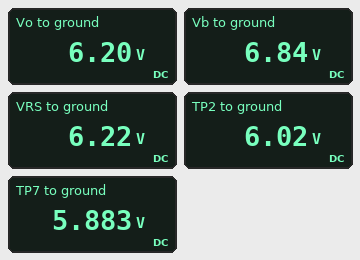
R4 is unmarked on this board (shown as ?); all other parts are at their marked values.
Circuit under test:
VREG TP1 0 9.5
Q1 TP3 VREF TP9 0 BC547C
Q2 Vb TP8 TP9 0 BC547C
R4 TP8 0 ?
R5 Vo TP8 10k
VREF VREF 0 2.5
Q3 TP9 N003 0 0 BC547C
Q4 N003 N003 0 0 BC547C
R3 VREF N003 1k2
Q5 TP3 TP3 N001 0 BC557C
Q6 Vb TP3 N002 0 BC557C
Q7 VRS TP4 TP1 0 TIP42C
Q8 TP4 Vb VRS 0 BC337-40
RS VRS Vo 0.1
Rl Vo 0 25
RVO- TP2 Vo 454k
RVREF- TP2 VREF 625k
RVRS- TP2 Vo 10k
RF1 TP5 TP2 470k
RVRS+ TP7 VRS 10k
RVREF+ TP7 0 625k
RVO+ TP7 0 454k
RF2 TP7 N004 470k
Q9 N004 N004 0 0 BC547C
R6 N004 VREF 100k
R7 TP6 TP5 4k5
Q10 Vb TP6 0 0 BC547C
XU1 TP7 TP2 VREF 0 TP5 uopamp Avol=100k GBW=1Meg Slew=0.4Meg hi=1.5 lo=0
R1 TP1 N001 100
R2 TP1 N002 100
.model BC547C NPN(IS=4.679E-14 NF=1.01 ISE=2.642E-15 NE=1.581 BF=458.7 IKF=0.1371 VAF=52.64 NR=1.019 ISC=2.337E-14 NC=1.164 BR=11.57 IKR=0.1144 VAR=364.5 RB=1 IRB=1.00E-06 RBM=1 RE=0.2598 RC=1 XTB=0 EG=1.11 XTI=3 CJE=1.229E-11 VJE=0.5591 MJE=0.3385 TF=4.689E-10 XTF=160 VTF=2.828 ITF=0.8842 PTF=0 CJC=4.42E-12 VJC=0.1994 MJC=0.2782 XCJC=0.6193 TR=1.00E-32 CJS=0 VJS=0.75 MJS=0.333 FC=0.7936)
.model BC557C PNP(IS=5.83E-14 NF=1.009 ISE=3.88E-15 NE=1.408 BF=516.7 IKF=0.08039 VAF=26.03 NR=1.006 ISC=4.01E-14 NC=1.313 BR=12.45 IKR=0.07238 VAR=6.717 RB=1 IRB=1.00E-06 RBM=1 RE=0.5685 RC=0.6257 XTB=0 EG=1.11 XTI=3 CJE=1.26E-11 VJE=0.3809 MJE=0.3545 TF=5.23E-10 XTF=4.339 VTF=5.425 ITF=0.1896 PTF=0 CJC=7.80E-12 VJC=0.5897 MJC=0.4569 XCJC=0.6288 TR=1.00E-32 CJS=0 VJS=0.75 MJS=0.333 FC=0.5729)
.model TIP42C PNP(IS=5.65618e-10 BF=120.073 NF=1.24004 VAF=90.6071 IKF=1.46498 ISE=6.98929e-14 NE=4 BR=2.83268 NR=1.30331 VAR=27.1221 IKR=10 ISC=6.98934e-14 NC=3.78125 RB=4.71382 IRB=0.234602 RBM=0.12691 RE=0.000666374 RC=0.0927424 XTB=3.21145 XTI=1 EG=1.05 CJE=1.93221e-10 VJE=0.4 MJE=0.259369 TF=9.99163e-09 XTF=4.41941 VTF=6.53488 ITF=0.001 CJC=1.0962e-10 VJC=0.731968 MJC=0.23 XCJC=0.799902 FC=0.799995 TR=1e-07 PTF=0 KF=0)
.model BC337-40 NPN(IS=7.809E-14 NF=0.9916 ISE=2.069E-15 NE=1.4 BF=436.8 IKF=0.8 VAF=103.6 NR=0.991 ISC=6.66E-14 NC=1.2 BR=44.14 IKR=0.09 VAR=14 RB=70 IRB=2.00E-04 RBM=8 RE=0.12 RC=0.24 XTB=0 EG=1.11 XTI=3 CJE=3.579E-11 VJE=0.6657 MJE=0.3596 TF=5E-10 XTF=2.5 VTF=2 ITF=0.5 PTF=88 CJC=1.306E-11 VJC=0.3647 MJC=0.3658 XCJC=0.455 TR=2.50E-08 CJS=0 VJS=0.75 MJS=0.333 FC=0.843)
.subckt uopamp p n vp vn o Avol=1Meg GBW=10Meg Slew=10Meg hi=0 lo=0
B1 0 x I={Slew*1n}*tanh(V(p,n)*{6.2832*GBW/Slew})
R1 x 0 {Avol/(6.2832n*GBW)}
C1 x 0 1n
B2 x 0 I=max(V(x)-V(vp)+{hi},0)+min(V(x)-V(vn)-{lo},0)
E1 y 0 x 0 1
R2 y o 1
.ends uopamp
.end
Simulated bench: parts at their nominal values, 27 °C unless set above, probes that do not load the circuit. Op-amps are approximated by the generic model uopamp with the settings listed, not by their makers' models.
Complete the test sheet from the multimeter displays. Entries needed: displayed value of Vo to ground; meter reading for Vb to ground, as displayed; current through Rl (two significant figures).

6.20 V
6.84 V
250 mA
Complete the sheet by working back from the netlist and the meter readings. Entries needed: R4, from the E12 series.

6.8 kΩ
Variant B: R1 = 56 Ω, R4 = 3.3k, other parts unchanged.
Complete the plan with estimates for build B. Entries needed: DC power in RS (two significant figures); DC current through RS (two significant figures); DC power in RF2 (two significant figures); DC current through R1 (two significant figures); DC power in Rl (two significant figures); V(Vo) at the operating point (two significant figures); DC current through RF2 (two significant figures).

12 mW
350 mA
130 µW
1.3 mA
3.1 W
8.8 V
17 µA
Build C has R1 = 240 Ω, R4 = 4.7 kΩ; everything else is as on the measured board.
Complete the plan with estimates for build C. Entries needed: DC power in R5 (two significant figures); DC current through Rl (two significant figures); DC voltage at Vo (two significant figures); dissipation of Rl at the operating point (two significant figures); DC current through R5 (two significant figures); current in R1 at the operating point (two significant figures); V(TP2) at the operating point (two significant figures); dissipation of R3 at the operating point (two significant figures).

2.9 mW
320 mA
7.9 V
2.5 W
540 µA
520 µA
7.7 V
2.9 mW
